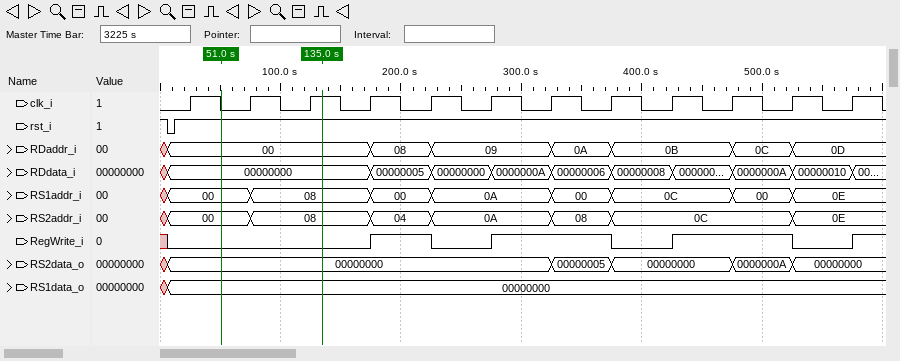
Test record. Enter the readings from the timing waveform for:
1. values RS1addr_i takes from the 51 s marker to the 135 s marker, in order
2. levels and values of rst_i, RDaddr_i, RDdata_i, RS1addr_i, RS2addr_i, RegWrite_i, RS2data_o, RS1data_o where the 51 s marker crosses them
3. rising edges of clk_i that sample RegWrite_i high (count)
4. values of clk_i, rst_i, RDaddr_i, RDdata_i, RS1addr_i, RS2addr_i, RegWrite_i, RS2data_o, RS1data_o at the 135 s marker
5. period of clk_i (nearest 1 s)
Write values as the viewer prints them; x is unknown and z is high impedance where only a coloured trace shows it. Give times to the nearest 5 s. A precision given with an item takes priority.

00, 08
rst_i=1, RDaddr_i=00, RDdata_i=00000000, RS1addr_i=00, RS2addr_i=00, RegWrite_i=0, RS2data_o=00000000, RS1data_o=00000000
5
clk_i=1, rst_i=1, RDaddr_i=00, RDdata_i=00000000, RS1addr_i=08, RS2addr_i=08, RegWrite_i=0, RS2data_o=00000000, RS1data_o=00000000
50 s
